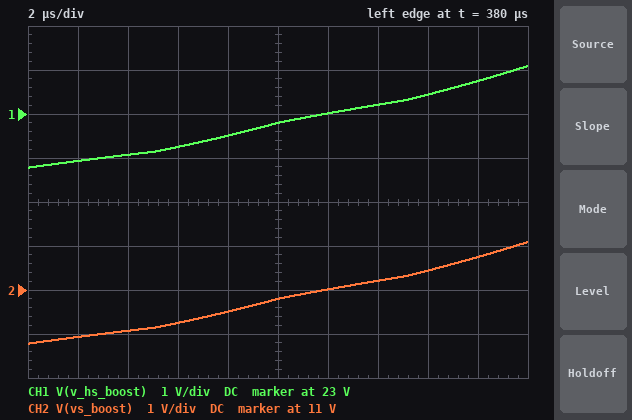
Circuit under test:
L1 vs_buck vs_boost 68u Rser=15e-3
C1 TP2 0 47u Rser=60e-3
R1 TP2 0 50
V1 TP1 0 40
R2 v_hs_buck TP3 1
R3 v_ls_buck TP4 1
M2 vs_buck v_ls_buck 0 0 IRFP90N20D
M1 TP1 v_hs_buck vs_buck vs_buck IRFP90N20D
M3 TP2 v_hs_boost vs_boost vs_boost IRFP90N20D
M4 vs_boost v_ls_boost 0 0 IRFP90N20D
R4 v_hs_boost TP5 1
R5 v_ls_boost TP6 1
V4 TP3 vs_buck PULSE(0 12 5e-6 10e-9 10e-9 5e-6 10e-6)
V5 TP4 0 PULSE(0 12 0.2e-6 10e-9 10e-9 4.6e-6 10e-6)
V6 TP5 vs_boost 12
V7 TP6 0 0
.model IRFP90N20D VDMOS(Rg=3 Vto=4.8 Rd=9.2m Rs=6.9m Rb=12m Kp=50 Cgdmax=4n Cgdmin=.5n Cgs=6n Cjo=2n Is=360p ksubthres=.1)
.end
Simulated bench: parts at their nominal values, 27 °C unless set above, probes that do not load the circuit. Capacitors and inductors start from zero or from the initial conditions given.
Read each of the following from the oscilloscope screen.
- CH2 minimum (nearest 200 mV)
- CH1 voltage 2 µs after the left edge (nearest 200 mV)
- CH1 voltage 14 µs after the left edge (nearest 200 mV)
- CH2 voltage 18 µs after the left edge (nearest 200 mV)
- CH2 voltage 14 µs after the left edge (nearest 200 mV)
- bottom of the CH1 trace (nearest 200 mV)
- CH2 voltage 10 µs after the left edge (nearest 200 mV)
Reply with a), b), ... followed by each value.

a) 9.8 V
b) 22.0 V
c) 23.2 V
d) 11.8 V
e) 11.2 V
f) 21.8 V
g) 10.8 V
